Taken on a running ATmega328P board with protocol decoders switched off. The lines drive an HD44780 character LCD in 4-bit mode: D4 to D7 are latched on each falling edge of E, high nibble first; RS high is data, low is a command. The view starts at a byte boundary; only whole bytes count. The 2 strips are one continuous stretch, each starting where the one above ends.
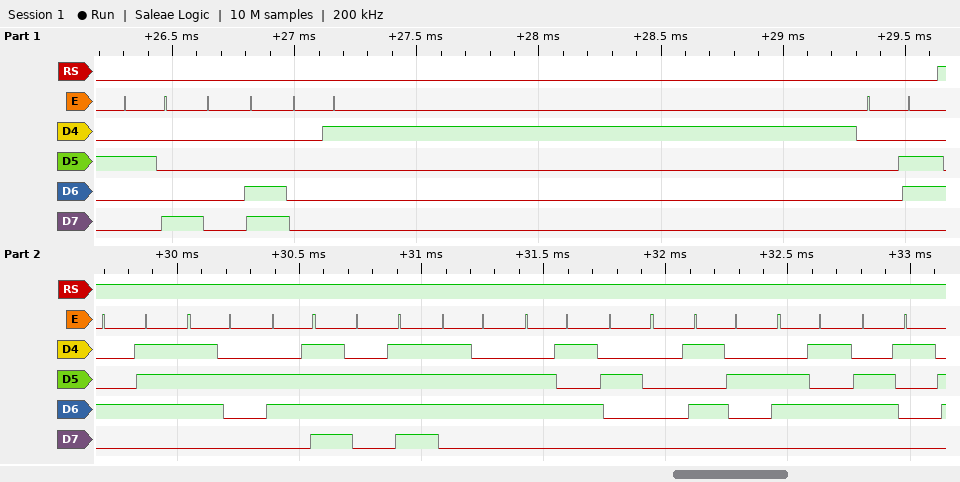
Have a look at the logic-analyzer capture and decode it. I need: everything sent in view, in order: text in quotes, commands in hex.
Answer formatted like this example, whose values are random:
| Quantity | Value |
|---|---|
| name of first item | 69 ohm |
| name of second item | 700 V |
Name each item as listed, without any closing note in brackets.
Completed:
| Quantity | Value |
|---|---|
| everything sent in view, in order: text in quotes, commands in hex | 0x28 0x0C 0x01 0x06 "Groove Rea" |
